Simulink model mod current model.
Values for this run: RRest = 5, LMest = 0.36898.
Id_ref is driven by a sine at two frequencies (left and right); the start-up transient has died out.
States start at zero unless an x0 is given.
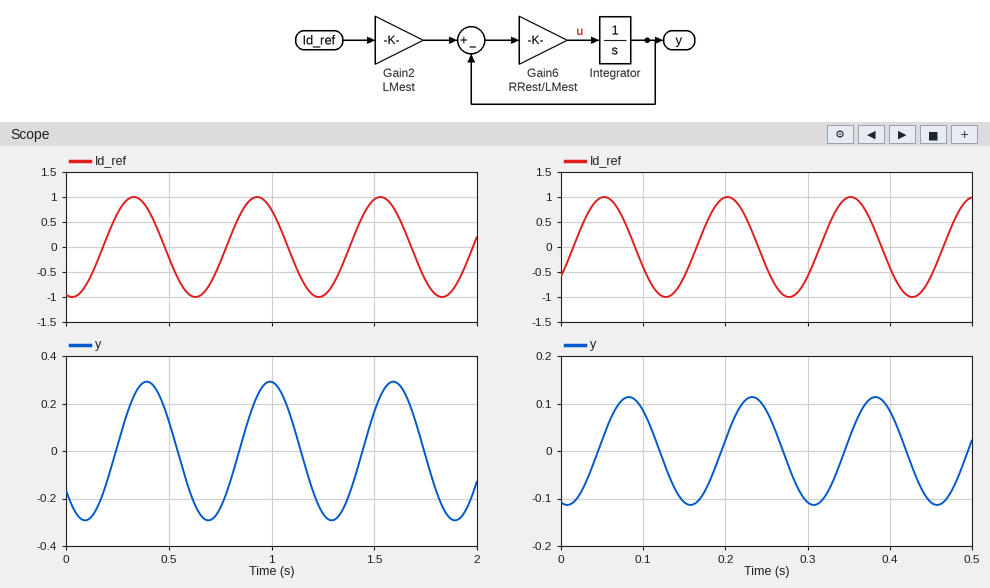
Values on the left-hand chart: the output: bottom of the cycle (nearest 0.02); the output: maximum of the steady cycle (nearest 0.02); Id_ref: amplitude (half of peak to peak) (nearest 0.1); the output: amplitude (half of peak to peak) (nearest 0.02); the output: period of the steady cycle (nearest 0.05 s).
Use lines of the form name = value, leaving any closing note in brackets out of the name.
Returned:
the output: bottom of the cycle = -0.30
the output: maximum of the steady cycle = 0.30
Id_ref: amplitude (half of peak to peak) = 1.0
the output: amplitude (half of peak to peak) = 0.30
the output: period of the steady cycle = 0.60 s
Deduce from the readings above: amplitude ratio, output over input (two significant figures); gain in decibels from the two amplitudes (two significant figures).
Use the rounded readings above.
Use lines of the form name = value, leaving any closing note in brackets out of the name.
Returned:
amplitude ratio, output over input = 0.30
gain in decibels from the two amplitudes = -10 dB
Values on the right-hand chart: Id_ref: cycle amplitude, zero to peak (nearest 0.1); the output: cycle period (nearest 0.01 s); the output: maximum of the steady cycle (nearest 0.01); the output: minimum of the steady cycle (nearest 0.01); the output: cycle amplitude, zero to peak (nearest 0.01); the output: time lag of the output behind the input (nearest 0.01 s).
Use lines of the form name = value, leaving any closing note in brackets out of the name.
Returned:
Id_ref: cycle amplitude, zero to peak = 1.0
the output: cycle period = 0.15 s
the output: maximum of the steady cycle = 0.11
the output: minimum of the steady cycle = -0.11
the output: cycle amplitude, zero to peak = 0.11
the output: time lag of the output behind the input = 0.03 s
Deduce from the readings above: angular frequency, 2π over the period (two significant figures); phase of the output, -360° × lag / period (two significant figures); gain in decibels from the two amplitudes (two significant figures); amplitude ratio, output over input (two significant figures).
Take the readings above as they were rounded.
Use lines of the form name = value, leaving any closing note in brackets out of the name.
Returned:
angular frequency, 2π over the period = 42 rad/s
phase of the output, -360° × lag / period = -72°
gain in decibels from the two amplitudes = -19 dB
amplitude ratio, output over input = 0.11
